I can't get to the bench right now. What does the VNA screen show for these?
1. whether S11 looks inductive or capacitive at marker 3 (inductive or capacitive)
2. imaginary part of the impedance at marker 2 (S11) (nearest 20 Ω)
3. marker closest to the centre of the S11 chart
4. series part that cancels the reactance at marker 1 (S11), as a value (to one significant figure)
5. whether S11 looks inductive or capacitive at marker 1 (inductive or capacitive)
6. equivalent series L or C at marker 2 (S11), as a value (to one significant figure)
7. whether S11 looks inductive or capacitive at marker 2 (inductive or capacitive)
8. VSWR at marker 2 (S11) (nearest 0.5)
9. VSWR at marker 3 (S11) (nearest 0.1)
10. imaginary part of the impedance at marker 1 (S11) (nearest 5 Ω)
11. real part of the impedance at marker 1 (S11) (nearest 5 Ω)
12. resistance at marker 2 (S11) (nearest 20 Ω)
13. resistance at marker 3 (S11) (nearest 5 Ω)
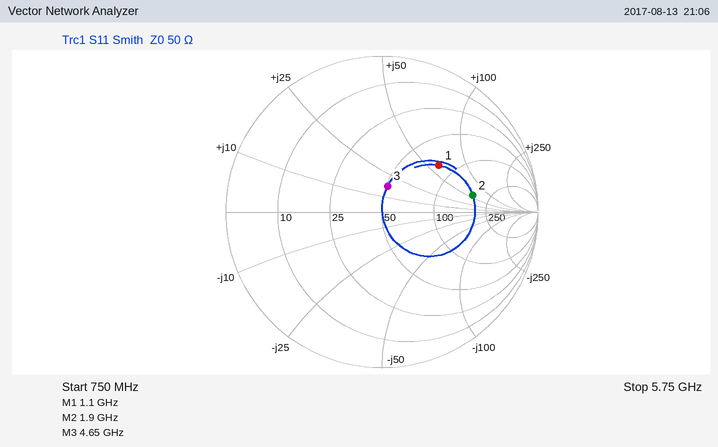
inductive
+60 Ω
marker 3
2 pF
inductive
5 nH
inductive
4.0
1.4
+60 Ω
80 Ω
180 Ω
50 Ω
